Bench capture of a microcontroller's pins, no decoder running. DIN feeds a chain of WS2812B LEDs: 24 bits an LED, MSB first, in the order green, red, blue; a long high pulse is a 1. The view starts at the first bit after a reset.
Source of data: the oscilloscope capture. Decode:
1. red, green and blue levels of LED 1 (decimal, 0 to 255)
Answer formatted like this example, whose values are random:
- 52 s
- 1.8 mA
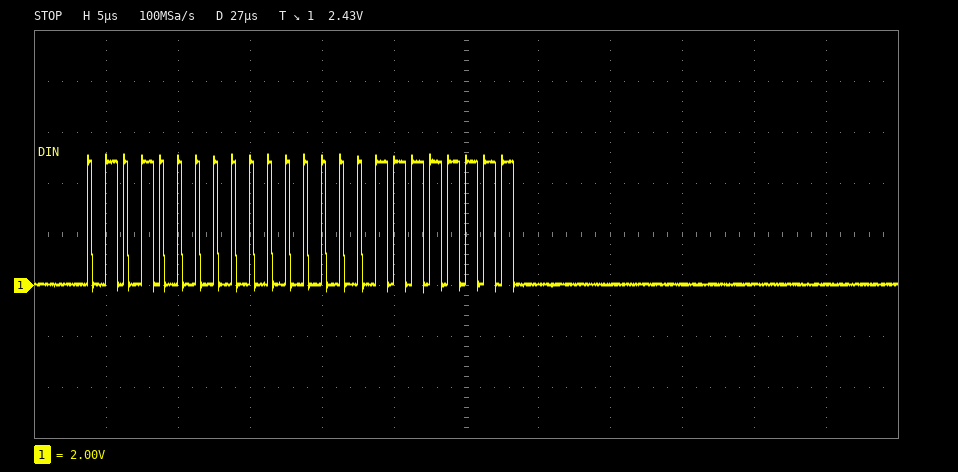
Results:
- 0, 80, 255
